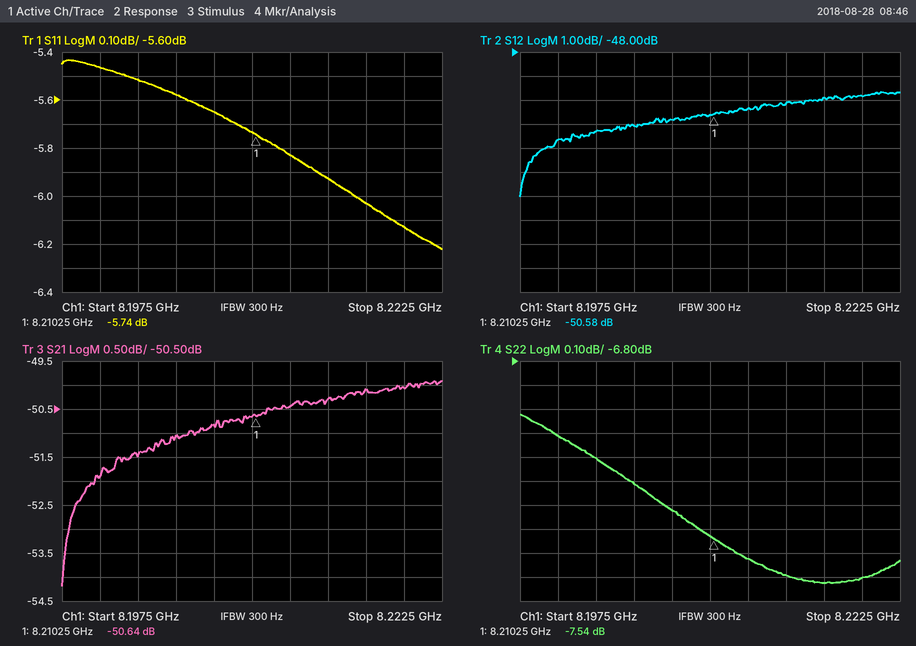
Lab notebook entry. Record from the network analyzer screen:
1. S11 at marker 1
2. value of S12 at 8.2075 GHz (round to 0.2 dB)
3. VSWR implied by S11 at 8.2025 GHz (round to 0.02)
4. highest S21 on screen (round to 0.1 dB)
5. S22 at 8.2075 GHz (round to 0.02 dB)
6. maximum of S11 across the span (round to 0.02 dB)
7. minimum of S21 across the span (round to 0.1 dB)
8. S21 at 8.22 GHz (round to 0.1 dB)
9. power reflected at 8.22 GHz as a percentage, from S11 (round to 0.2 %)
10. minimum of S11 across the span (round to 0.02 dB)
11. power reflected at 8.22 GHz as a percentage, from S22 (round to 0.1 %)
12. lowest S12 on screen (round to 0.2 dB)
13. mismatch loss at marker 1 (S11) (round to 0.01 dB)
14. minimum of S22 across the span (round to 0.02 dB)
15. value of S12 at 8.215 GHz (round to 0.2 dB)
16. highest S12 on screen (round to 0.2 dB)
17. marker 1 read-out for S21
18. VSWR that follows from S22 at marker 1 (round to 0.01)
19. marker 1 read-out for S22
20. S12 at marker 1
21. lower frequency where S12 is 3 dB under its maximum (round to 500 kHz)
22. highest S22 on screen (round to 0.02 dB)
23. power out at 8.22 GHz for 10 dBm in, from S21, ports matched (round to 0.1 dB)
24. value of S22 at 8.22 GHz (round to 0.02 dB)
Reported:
-5.74 dB
-50.8 dB
3.26
-49.9 dB
-7.42 dB
-5.44 dB
-54.2 dB
-50.1 dB
24.4 %
-6.22 dB
17.0 %
-54.0 dB
1.35 dB
-7.72 dB
-50.2 dB
-49.6 dB
-50.64 dB
2.45
-7.54 dB
-50.58 dB
8.1980 GHz
-7.02 dB
-40.1 dBm
-7.70 dB
